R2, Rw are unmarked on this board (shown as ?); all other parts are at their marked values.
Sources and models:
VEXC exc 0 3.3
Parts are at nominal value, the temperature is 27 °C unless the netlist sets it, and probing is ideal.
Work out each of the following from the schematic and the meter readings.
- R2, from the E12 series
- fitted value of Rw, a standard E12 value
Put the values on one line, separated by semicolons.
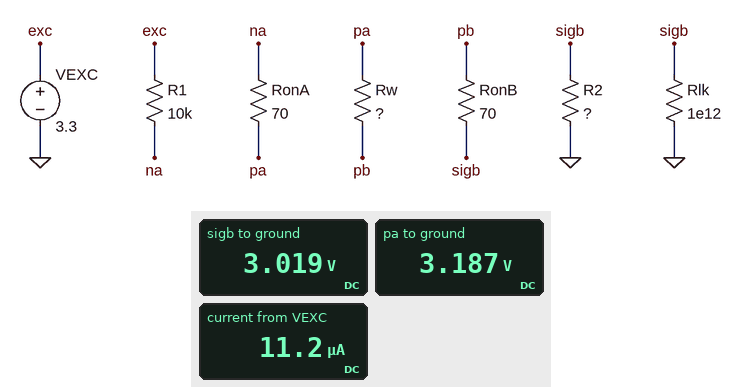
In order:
270 kΩ; 15 kΩ
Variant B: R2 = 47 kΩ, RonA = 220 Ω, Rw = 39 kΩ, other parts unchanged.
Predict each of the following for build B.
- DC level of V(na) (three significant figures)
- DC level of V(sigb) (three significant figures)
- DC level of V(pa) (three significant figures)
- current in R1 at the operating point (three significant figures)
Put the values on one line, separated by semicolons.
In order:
2.96 V; 1.61 V; 2.95 V; 34.3 µA
